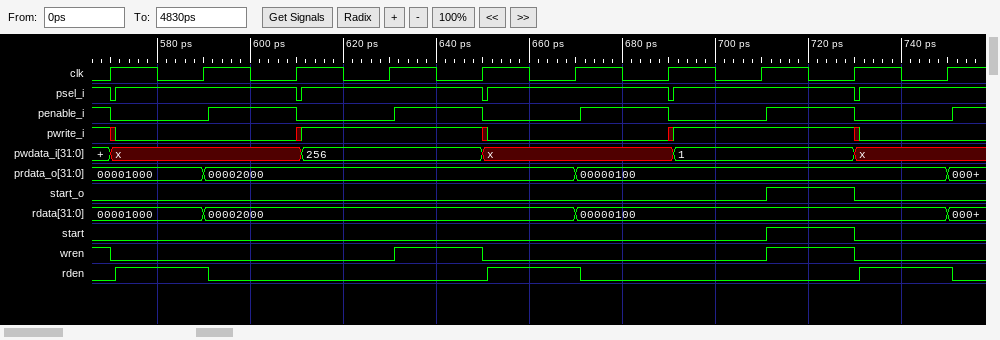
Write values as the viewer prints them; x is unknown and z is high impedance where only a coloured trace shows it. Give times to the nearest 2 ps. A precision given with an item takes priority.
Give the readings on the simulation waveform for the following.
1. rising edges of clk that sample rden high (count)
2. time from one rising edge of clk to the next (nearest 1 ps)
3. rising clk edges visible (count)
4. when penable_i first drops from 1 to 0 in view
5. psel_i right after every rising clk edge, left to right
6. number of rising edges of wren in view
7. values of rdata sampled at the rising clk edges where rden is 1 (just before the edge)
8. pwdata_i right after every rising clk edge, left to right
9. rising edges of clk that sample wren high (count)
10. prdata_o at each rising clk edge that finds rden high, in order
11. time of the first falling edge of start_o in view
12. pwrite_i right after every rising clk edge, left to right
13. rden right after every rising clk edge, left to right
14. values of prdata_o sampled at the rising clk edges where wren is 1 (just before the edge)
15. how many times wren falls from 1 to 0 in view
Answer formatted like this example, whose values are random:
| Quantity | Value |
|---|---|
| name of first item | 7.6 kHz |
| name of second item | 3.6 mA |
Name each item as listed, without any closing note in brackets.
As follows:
| Quantity | Value |
|---|---|
| rising edges of clk that sample rden high | 3 |
| time from one rising edge of clk to the next | 20 ps |
| rising clk edges visible | 10 |
| when penable_i first drops from 1 to 0 in view | 570 ps |
| psel_i right after every rising clk edge, left to right | 0 1 0 1 0 1 0 1 0 1 |
| number of rising edges of wren in view | 2 |
| values of rdata sampled at the rising clk edges where rden is 1 | 00001000, 00002000, 00000100 |
| pwdata_i right after every rising clk edge, left to right | x, x, x, 256, x, x, x, 1, x, x |
| rising edges of clk that sample wren high | 3 |
| prdata_o at each rising clk edge that finds rden high, in order | 00001000, 00002000, 00000100 |
| time of the first falling edge of start_o in view | 730 ps |
| pwrite_i right after every rising clk edge, left to right | x 0 x 1 x 0 x 1 x 0 |
| rden right after every rising clk edge, left to right | 0 1 0 0 0 1 0 0 0 1 |
| values of prdata_o sampled at the rising clk edges where wren is 1 | 00001000, 00002000, 00000100 |
| how many times wren falls from 1 to 0 in view | 3 |
